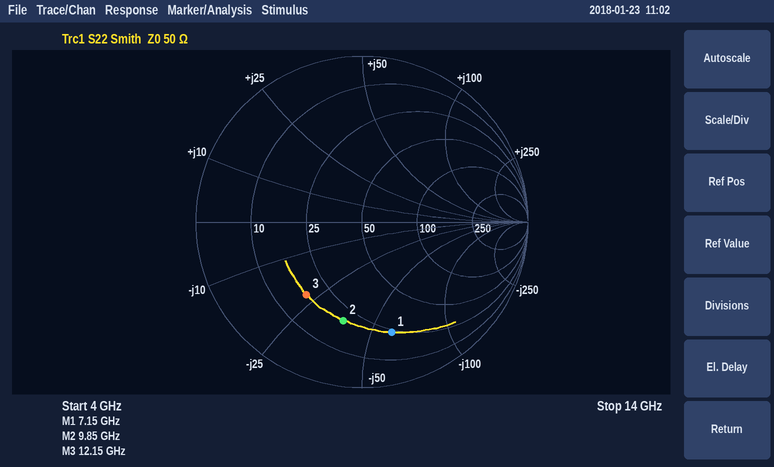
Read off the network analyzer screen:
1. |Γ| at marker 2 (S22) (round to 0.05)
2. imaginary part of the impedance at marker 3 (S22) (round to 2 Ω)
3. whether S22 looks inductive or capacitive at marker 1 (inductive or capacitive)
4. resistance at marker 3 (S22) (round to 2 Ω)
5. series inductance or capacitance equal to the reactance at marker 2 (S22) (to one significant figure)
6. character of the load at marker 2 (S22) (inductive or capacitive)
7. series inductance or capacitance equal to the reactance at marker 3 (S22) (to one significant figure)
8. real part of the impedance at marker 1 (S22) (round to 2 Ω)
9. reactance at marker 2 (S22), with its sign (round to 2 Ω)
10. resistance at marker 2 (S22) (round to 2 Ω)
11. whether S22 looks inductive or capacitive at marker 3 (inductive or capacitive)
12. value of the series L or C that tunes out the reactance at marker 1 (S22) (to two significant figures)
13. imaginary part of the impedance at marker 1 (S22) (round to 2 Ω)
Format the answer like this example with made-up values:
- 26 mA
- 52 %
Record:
- 0.60
- -22 Ω
- capacitive
- 18 Ω
- 400 fF
- capacitive
- 600 fF
- 24 Ω
- -38 Ω
- 20 Ω
- capacitive
- 1.3 nH
- -60 Ω
